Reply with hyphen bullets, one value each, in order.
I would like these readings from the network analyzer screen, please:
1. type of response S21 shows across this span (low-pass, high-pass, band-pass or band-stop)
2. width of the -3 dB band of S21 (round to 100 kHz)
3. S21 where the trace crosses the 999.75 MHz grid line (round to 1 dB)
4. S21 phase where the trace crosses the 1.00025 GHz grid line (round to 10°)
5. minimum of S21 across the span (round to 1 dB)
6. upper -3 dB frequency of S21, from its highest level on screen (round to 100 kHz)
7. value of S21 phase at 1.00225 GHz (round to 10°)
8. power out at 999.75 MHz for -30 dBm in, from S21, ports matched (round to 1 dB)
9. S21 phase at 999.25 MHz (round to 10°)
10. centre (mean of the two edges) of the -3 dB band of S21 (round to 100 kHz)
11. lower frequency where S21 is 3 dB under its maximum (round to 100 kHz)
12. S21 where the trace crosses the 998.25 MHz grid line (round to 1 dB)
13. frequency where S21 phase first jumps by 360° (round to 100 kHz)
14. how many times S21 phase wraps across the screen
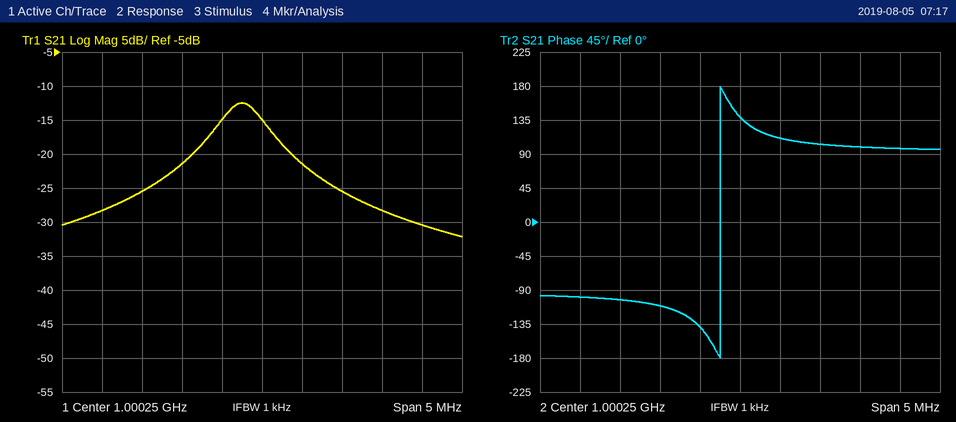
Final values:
- band-pass
- 600 kHz
- -15 dB
- 140°
- -32 dB
- 1.0003 GHz
- 100°
- -45 dBm
- -110°
- 1.0000 GHz
- 999.7 MHz
- -28 dB
- 1.0000 GHz
- 1
